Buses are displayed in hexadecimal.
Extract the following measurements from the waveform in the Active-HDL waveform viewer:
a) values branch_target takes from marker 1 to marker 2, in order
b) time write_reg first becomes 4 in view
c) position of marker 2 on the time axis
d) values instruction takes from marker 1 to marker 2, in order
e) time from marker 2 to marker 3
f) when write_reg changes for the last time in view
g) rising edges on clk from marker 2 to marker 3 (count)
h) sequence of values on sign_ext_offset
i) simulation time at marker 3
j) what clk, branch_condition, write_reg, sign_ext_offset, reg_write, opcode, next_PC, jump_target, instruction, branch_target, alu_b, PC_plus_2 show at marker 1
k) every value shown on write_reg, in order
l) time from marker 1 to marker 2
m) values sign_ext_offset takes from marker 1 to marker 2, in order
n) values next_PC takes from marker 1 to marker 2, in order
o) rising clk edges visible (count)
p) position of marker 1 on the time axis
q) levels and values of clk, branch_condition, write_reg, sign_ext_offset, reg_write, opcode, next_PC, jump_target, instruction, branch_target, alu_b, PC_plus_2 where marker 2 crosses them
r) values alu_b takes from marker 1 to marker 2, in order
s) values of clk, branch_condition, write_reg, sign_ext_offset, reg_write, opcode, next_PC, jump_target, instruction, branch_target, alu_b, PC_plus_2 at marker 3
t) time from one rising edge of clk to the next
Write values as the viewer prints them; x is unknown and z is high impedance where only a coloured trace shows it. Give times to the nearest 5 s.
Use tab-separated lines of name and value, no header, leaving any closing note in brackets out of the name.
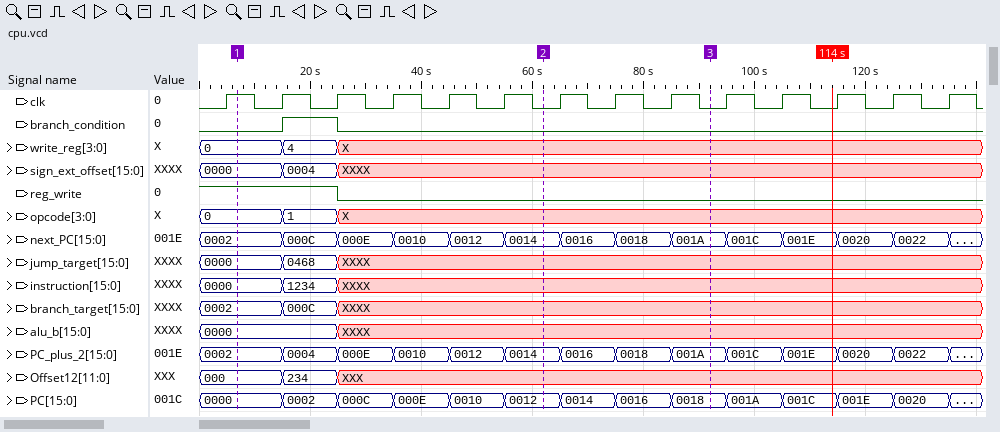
values branch_target takes from marker 1 to marker 2, in order	0002, 000C, XXXX
time write_reg first becomes 4 in view	15 s
position of marker 2 on the time axis	60 s
values instruction takes from marker 1 to marker 2, in order	0000, 1234, XXXX
time from marker 2 to marker 3	30 s
when write_reg changes for the last time in view	25 s
rising edges on clk from marker 2 to marker 3	3
sequence of values on sign_ext_offset	0000, 0004, XXXX
simulation time at marker 3	90 s
what clk, branch_condition, write_reg, sign_ext_offset, reg_write, opcode, next_PC, jump_target, instruction, branch_target, alu_b, PC_plus_2 show at marker 1	clk=1, branch_condition=0, write_reg=0, sign_ext_offset=0000, reg_write=1, opcode=0, next_PC=0002, jump_target=0000, instruction=0000, branch_target=0002, alu_b=0000, PC_plus_2=0002
every value shown on write_reg, in order	0, 4, X
time from marker 1 to marker 2	55 s
values sign_ext_offset takes from marker 1 to marker 2, in order	0000, 0004, XXXX
values next_PC takes from marker 1 to marker 2, in order	0002, 000C, 000E, 0010, 0012, 0014
rising clk edges visible	14
position of marker 1 on the time axis	5 s
levels and values of clk, branch_condition, write_reg, sign_ext_offset, reg_write, opcode, next_PC, jump_target, instruction, branch_target, alu_b, PC_plus_2 where marker 2 crosses them	clk=0, branch_condition=0, write_reg=X, sign_ext_offset=XXXX, reg_write=0, opcode=X, next_PC=0014, jump_target=XXXX, instruction=XXXX, branch_target=XXXX, alu_b=XXXX, PC_plus_2=0014
values alu_b takes from marker 1 to marker 2, in order	0000, XXXX
values of clk, branch_condition, write_reg, sign_ext_offset, reg_write, opcode, next_PC, jump_target, instruction, branch_target, alu_b, PC_plus_2 at marker 3	clk=0, branch_condition=0, write_reg=X, sign_ext_offset=XXXX, reg_write=0, opcode=X, next_PC=001A, jump_target=XXXX, instruction=XXXX, branch_target=XXXX, alu_b=XXXX, PC_plus_2=001A
time from one rising edge of clk to the next	10 s
